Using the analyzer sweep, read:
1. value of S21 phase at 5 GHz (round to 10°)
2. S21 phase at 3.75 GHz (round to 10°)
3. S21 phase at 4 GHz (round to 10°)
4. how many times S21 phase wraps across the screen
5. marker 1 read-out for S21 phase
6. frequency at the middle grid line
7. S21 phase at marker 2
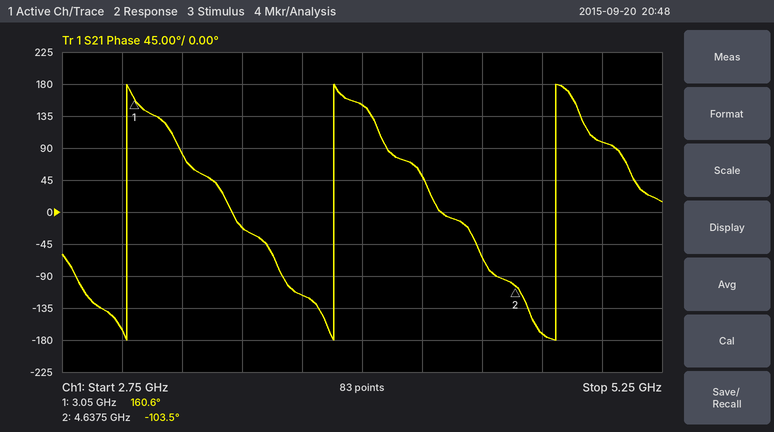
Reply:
100°
-120°
150°
3
160.6°
4 GHz
-103.5°
